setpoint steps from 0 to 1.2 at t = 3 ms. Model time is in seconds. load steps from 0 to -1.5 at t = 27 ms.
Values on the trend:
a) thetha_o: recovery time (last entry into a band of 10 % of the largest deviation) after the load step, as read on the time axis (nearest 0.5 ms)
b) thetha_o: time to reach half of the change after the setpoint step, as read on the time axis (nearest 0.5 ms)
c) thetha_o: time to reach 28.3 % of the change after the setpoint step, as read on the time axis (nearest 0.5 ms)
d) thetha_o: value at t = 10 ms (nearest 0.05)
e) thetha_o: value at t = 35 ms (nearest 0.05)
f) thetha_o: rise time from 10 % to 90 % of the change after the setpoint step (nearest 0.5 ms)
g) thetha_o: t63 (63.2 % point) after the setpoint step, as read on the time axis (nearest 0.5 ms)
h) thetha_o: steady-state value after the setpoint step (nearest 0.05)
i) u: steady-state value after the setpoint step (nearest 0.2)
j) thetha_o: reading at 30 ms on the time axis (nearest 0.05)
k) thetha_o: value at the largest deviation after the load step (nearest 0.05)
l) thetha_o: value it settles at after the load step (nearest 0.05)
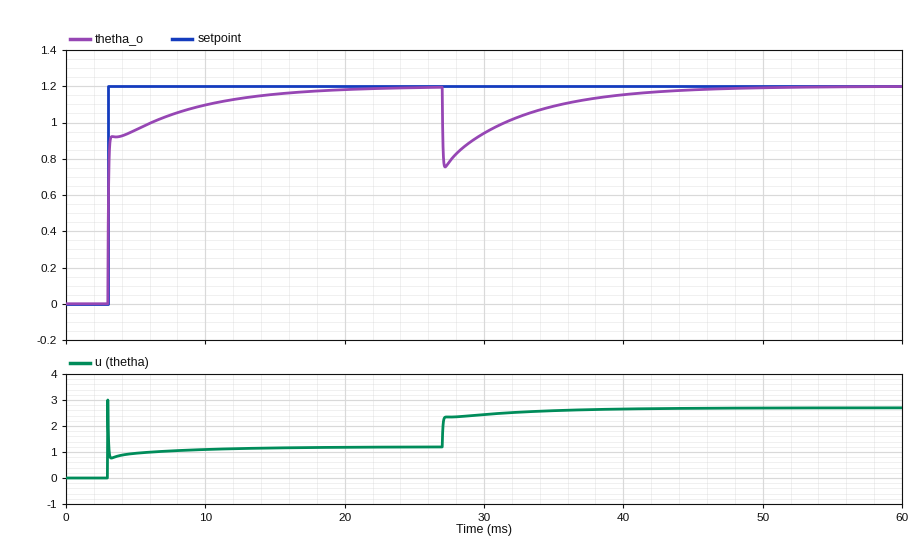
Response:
40.5 ms
3.0 ms
3.0 ms
1.10
1.10
6.0 ms
3.0 ms
1.20
1.2
0.95
0.75
1.20
